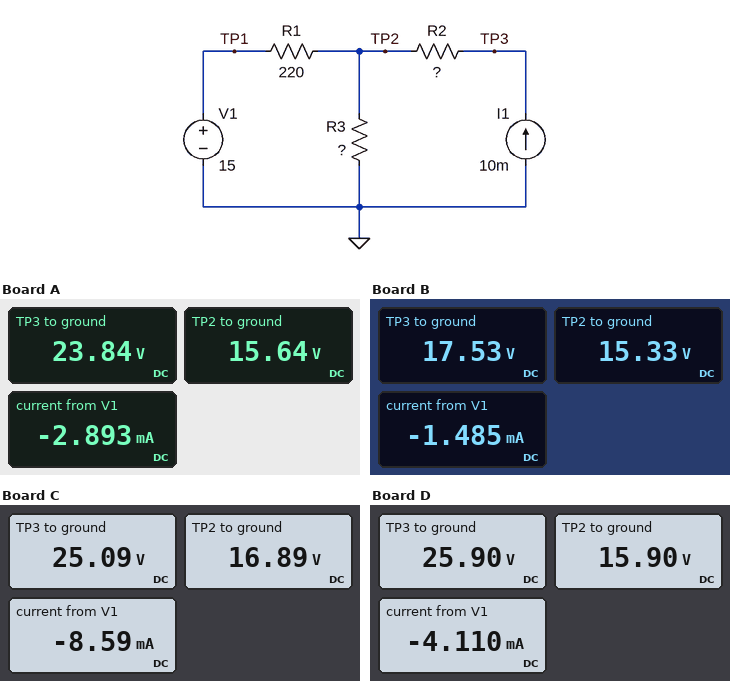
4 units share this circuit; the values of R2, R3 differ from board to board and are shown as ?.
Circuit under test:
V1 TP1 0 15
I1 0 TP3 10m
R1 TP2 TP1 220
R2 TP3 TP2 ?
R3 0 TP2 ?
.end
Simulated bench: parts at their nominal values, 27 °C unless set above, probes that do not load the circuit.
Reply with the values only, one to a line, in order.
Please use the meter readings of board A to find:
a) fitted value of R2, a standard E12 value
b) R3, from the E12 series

820 Ω
2.2 kΩ
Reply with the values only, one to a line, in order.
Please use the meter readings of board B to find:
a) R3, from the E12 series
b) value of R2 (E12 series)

1.8 kΩ
220 Ω
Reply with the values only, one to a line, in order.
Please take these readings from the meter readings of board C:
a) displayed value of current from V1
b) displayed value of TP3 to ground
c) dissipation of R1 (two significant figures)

-8.59 mA
25.09 V
16 mW
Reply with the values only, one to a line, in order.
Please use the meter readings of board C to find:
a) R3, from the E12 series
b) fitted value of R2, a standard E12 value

12 kΩ
820 Ω
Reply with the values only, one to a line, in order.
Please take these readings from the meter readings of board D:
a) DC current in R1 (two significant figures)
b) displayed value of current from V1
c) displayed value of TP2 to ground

4.1 mA
-4.110 mA
15.90 V
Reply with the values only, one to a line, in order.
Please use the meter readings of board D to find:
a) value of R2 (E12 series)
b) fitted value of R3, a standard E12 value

1 kΩ
2.7 kΩ
